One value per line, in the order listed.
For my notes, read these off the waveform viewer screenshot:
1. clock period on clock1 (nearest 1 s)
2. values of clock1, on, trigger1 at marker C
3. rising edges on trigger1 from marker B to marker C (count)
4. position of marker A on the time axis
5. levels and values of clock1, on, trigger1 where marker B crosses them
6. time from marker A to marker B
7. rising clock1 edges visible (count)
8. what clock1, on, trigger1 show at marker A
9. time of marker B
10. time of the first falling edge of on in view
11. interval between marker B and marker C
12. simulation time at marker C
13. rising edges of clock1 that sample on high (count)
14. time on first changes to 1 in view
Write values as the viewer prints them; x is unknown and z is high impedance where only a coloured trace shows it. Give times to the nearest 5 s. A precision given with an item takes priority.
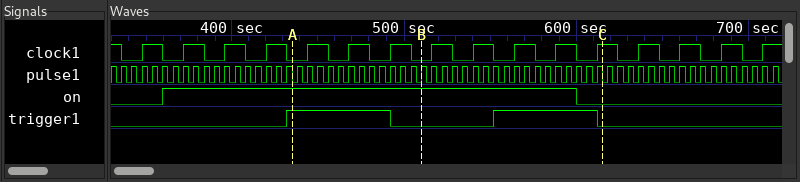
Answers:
24 s
clock1=1, on=0, trigger1=0
1
435 s
clock1=0, on=1, trigger1=0
75 s
16
clock1=0, on=1, trigger1=1
510 s
600 s
105 s
615 s
10
360 s
